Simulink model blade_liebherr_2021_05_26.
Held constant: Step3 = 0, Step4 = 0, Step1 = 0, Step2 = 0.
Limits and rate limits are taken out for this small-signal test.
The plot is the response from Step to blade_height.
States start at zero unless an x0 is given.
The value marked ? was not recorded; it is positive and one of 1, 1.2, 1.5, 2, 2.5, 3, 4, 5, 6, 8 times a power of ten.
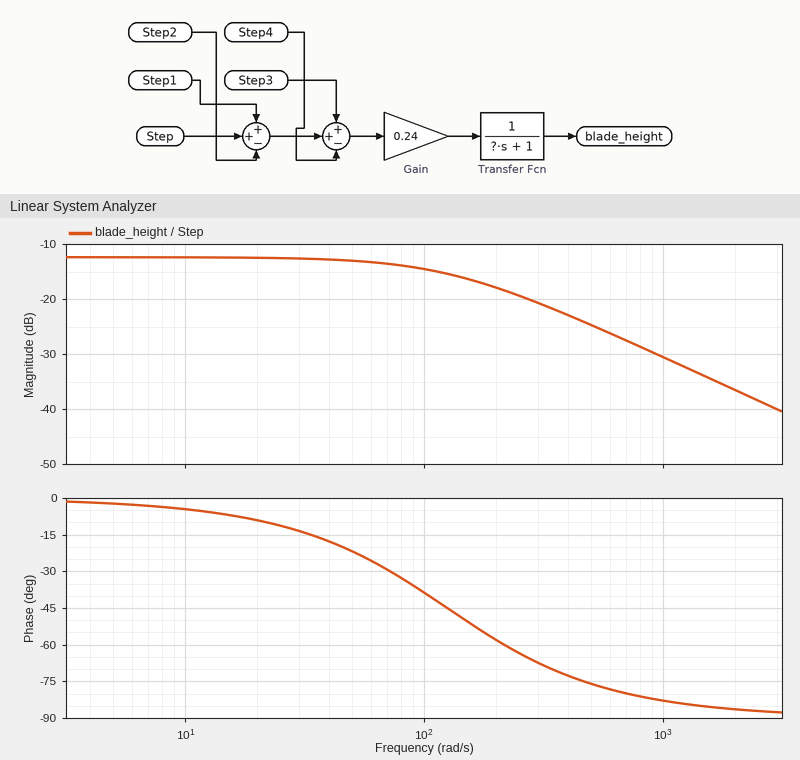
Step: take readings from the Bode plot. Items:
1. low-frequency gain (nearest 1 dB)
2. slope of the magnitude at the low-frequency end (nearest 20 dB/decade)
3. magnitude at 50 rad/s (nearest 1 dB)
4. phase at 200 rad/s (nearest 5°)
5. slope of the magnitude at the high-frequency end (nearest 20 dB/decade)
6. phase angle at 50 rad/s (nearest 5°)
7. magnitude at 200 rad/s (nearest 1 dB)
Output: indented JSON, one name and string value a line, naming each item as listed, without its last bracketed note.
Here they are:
{
  "low-frequency gain": "-12 dB",
  "slope of the magnitude at the low-frequency end": "0 dB/decade",
  "magnitude at 50 rad/s": "-13 dB",
  "phase at 200 rad/s": "-60°",
  "slope of the magnitude at the high-frequency end": "-20 dB/decade",
  "phase angle at 50 rad/s": "-20°",
  "magnitude at 200 rad/s": "-18 dB"
}
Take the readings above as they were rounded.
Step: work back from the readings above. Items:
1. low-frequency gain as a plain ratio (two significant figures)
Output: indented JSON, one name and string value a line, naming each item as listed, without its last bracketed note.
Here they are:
{
  "low-frequency gain as a plain ratio": "0.25"
}
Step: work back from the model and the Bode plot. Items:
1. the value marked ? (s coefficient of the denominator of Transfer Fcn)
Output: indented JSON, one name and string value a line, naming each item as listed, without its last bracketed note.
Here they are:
{
  "the value marked ?": "0.008"
}
